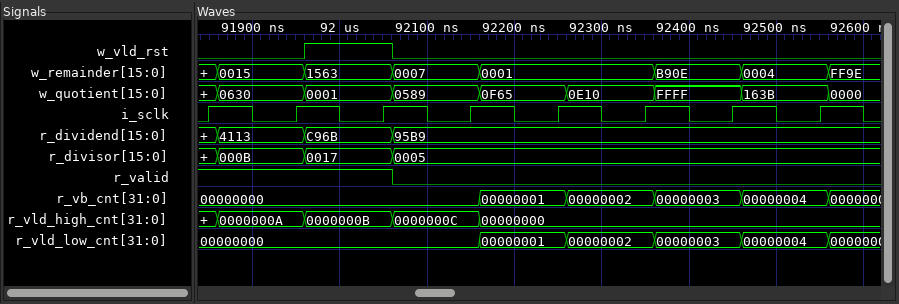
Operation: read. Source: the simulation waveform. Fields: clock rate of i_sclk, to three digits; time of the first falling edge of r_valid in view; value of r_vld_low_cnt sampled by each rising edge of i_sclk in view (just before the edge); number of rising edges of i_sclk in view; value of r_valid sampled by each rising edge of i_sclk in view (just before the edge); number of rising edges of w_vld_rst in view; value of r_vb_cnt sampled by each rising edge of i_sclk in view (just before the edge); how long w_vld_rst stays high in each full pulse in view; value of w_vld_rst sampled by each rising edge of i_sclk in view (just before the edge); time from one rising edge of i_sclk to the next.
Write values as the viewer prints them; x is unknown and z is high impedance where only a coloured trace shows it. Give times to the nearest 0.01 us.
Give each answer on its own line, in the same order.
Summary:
10.0 MHz
92.06 us
00000000, 00000000, 00000000, 00000000, 00000001, 00000002, 00000003, 00000004
8
1 1 1 0 0 0 0 0
1
00000000, 00000000, 00000000, 00000000, 00000001, 00000002, 00000003, 00000004
0.1 us
0 0 1 0 0 0 0 0
0.1 us
